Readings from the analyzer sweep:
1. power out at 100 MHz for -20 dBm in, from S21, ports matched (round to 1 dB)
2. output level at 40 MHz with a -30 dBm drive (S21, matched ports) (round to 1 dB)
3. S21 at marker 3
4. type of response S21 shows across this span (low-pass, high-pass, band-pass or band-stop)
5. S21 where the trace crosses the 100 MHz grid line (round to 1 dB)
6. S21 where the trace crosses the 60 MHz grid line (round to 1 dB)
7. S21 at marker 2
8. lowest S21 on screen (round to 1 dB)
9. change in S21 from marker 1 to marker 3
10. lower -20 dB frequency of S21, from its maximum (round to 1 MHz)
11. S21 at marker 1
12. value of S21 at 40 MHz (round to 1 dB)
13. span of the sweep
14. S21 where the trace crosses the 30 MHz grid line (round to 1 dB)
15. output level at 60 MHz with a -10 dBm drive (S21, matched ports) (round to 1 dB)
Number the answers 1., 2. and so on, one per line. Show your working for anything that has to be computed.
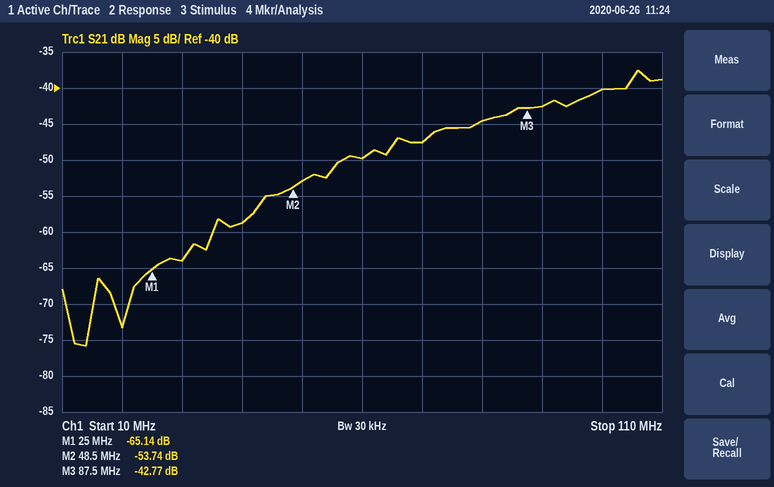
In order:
1. -20 dBm + (-40 dB) = -60 dBm
2. -30 dBm + (-59 dB) = -89 dBm
3. -42.77 dB
4. high-pass
5. -40 dB
6. -50 dB
7. -53.74 dB
8. -76 dB
9. -42.77 − (-65.14) = 22.37 dB
10. 42 MHz
11. -65.14 dB
12. -59 dB
13. 100 MHz
14. -64 dB
15. -10 dBm + (-50 dB) = -60 dBm
